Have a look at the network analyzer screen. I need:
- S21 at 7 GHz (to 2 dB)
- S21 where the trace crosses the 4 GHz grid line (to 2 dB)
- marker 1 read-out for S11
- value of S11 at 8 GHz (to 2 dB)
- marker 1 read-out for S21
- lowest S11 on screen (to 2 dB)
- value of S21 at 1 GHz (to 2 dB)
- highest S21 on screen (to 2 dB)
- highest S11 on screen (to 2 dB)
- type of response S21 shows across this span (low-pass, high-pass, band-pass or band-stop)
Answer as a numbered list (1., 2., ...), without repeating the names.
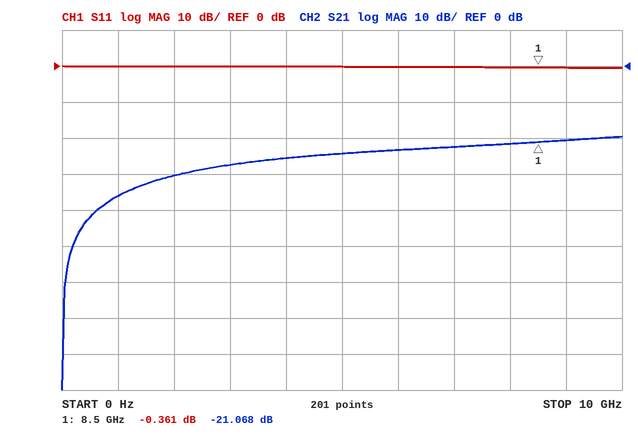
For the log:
1. -22 dB
2. -26 dB
3. -0.361 dB
4. 0 dB
5. -21.068 dB
6. 0 dB
7. -36 dB
8. -20 dB
9. 0 dB
10. high-pass
